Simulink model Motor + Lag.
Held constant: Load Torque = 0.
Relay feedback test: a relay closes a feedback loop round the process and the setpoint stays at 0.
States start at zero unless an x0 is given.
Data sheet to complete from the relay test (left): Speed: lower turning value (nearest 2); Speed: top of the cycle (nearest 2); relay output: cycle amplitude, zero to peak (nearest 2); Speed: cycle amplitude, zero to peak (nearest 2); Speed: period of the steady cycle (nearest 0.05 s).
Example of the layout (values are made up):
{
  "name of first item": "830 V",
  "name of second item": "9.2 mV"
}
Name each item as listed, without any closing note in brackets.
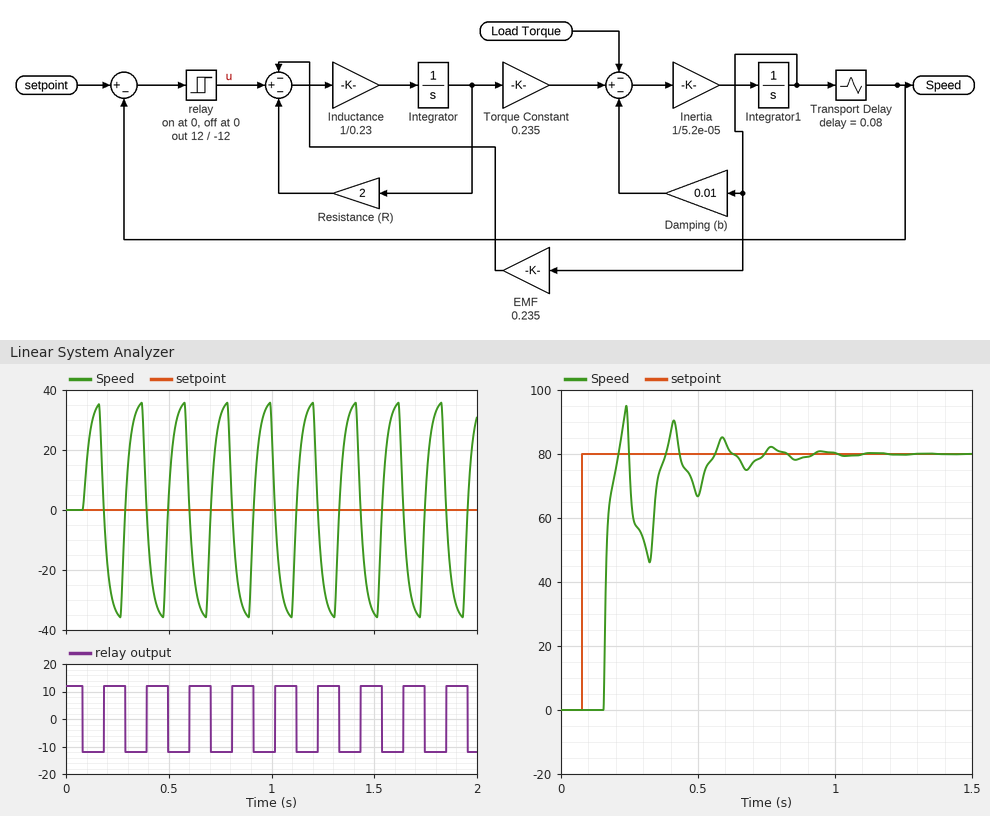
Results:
{
  "Speed: lower turning value": "-36",
  "Speed: top of the cycle": "36",
  "relay output: cycle amplitude, zero to peak": "12",
  "Speed: cycle amplitude, zero to peak": "36",
  "Speed: period of the steady cycle": "0.20 s"
}
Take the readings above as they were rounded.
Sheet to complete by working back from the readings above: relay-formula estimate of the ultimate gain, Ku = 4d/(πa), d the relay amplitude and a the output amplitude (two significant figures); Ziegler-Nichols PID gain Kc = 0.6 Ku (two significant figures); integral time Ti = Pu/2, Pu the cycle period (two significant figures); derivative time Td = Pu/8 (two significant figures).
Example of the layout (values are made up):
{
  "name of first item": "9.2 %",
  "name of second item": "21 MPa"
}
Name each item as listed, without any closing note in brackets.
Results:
{
  "relay-formula estimate of the ultimate gain, Ku = 4d/(πa), d the relay amplitude and a the output amplitude": "0.42",
  "Ziegler-Nichols PID gain Kc = 0.6 Ku": "0.25",
  "integral time Ti = Pu/2, Pu the cycle period": "0.10 s",
  "derivative time Td = Pu/8": "0.025 s"
}
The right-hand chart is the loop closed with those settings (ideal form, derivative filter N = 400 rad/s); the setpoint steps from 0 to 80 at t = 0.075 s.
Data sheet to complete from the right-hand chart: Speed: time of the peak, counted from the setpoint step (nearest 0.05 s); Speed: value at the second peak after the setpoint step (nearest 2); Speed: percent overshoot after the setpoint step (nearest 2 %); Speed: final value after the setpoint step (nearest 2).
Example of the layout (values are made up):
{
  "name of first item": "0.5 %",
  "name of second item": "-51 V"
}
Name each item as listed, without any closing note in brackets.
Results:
{
  "Speed: time of the peak, counted from the setpoint step": "0.15 s",
  "Speed: value at the second peak after the setpoint step": "90",
  "Speed: percent overshoot after the setpoint step": "18 %",
  "Speed: final value after the setpoint step": "80"
}
